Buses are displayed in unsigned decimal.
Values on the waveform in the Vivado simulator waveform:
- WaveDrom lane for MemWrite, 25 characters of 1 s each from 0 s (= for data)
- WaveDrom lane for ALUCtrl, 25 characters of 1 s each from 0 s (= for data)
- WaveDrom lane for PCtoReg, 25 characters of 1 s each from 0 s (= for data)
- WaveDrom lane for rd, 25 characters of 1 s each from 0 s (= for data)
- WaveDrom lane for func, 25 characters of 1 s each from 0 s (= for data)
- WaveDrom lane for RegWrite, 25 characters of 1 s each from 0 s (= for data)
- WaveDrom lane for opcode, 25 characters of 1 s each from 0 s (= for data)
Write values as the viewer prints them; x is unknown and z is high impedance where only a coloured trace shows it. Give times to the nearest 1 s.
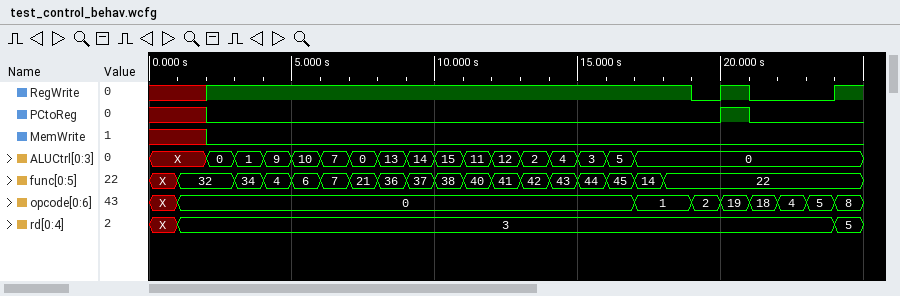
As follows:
{name: 'MemWrite', wave: 'x.0......................'}
{name: 'ALUCtrl', wave: 'x.================.......', data: '0 1 9 10 7 0 13 14 15 11 12 2 4 3 5 0'}
{name: 'PCtoReg', wave: 'x.0.................10...'}
{name: 'rd', wave: 'x=......................=', data: '3 5'}
{name: 'func', wave: 'x=.================......', data: '32 34 4 6 7 21 36 37 38 40 41 42 43 44 45 14 22'}
{name: 'RegWrite', wave: 'x.1................010..1'}
{name: 'opcode', wave: 'x=...............=.======', data: '0 1 2 19 18 4 5 8'}
